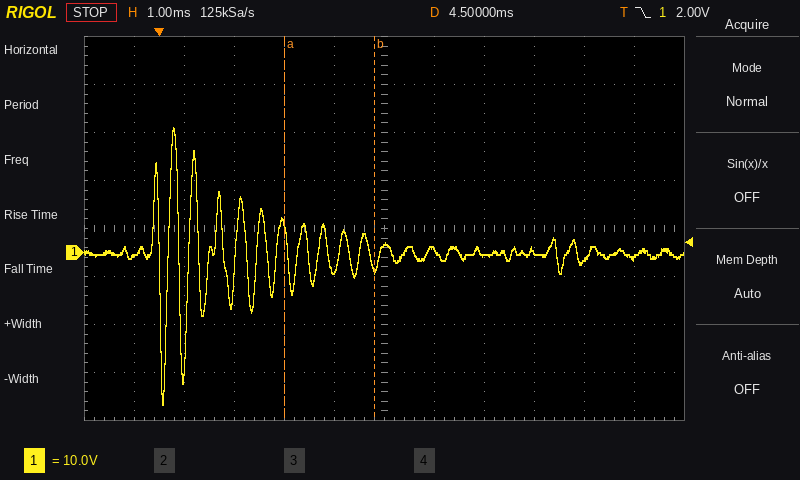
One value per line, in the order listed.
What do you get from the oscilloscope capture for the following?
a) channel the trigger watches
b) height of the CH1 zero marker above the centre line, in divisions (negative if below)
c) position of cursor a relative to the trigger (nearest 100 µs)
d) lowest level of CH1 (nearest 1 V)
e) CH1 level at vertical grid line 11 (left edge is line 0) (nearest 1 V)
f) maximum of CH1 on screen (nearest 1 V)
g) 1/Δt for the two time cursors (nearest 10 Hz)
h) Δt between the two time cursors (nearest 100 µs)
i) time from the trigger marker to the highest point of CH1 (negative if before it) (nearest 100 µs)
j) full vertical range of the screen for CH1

CH1
-0.5 div
+2.5 ms
-32 V
-1 V
26 V
560 Hz
1.8 ms
+300 µs
80 V
